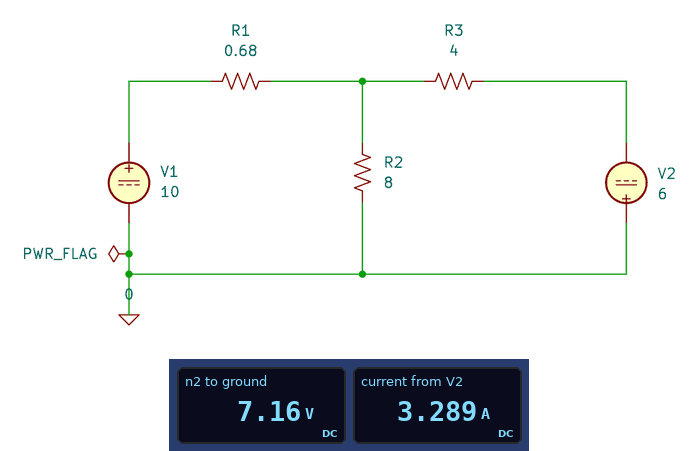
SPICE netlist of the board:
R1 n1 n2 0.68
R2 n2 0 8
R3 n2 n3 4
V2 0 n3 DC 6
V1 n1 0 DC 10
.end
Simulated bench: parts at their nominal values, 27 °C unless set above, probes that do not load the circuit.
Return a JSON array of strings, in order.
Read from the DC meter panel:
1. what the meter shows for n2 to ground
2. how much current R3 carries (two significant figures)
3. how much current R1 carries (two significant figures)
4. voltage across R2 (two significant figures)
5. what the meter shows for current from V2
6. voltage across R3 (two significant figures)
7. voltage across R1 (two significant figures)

["7.16 V", "3.3 A", "4.2 A", "7.2 V", "3.289 A", "13 V", "2.8 V"]
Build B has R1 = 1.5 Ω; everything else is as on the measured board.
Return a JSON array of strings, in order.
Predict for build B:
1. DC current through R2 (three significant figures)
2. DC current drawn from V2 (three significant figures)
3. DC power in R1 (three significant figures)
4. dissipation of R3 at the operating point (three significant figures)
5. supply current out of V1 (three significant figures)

["620 mA", "2.74 A", "16.9 W", "30.0 W", "3.36 A"]
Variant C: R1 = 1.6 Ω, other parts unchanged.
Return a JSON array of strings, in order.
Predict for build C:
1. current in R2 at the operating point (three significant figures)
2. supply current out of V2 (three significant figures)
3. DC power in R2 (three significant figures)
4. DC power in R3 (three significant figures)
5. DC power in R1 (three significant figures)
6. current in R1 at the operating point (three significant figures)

["594 mA", "2.69 A", "2.82 W", "28.9 W", "17.2 W", "3.28 A"]
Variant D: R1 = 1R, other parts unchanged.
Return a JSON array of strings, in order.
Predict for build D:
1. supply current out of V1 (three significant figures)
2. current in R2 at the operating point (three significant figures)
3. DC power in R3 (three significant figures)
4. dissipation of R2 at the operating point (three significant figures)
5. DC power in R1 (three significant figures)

["3.82 A", "773 mA", "37.1 W", "4.78 W", "14.6 W"]
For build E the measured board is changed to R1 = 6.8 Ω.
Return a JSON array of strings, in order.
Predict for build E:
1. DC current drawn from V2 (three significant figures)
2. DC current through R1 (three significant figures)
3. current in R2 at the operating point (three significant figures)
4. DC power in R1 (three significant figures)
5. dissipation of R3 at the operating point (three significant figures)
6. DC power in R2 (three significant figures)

["1.49 A", "1.48 A", "7.04 mA", "14.9 W", "8.83 W", "397 µW"]
